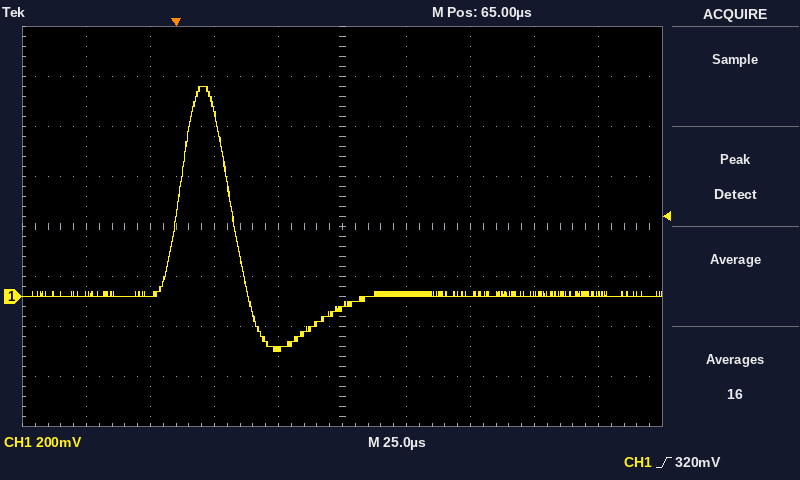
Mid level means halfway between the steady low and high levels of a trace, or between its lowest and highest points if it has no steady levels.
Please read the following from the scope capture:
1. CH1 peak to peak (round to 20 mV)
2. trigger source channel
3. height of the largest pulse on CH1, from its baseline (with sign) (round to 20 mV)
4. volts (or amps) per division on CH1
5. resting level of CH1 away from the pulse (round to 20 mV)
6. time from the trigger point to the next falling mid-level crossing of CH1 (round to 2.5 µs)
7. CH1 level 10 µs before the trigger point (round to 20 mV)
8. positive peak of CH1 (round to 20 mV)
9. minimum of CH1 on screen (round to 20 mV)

1.06 V
CH1
+840 mV
200 mV
0 mV
22.5 µs
0 mV
840 mV
-220 mV
